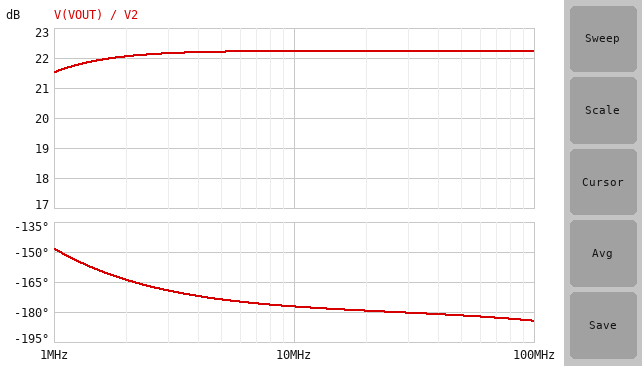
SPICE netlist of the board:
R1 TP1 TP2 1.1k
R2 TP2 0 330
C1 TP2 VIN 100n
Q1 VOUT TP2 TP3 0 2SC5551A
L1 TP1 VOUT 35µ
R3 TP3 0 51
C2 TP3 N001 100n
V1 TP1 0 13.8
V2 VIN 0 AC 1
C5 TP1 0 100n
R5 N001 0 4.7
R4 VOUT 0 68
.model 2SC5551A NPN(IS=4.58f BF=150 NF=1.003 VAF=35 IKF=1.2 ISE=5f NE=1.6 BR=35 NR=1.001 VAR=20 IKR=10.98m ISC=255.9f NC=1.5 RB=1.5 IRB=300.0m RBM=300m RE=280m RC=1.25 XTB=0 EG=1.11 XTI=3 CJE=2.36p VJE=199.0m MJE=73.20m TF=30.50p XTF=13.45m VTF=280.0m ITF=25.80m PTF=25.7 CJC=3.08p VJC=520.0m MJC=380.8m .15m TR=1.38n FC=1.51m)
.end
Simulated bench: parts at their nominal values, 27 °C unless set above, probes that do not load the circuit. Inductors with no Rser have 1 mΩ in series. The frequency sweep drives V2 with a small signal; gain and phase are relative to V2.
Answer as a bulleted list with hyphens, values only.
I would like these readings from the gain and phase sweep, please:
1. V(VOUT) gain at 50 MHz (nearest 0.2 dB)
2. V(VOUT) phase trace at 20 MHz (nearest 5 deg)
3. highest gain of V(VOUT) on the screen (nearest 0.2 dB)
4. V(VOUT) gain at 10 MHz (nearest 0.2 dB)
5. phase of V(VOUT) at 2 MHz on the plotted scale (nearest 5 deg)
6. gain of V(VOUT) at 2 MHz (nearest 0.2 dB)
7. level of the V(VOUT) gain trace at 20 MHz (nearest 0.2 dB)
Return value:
- 22.2 dB
- -180 deg
- 22.2 dB
- 22.2 dB
- -165 deg
- 22.0 dB
- 22.2 dB
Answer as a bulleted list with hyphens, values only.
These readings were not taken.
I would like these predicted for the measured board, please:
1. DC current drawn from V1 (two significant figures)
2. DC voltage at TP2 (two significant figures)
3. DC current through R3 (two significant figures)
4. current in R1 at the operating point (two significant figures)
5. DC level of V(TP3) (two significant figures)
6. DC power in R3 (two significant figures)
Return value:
- 260 mA
- 3.1 V
- 46 mA
- 9.7 mA
- 2.3 V
- 110 mW
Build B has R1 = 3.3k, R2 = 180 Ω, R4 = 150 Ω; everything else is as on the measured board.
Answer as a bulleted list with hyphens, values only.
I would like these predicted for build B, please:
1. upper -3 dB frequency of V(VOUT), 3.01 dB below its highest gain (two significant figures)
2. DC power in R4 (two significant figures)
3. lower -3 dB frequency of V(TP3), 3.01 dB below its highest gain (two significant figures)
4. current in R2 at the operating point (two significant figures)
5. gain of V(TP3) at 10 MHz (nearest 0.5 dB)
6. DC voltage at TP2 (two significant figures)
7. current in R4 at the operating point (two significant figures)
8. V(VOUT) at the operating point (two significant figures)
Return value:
- 1.3 GHz
- 1.3 W
- 7.6 kHz
- 4.0 mA
- -18.0 dB
- 710 mV
- 92 mA
- 14 V
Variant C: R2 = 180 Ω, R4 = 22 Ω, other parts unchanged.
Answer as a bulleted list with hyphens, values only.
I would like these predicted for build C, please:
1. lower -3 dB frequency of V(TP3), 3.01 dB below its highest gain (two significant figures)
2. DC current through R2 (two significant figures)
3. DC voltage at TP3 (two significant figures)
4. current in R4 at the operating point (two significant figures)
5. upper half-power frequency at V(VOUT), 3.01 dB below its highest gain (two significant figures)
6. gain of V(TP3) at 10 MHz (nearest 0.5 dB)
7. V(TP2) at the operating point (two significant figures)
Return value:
- 9.9 kHz
- 11 mA
- 1.2 V
- 630 mA
- 4.7 GHz
- -2.5 dB
- 1.9 V
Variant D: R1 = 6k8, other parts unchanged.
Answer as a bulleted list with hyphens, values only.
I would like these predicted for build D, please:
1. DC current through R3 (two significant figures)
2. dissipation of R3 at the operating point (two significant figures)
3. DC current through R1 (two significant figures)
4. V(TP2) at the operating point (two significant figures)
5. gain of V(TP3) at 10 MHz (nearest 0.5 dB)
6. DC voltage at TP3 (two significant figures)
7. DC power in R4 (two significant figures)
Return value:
- 200 µA
- 2.1 µW
- 1.9 mA
- 640 mV
- -30.0 dB
- 10 mV
- 2.8 W
